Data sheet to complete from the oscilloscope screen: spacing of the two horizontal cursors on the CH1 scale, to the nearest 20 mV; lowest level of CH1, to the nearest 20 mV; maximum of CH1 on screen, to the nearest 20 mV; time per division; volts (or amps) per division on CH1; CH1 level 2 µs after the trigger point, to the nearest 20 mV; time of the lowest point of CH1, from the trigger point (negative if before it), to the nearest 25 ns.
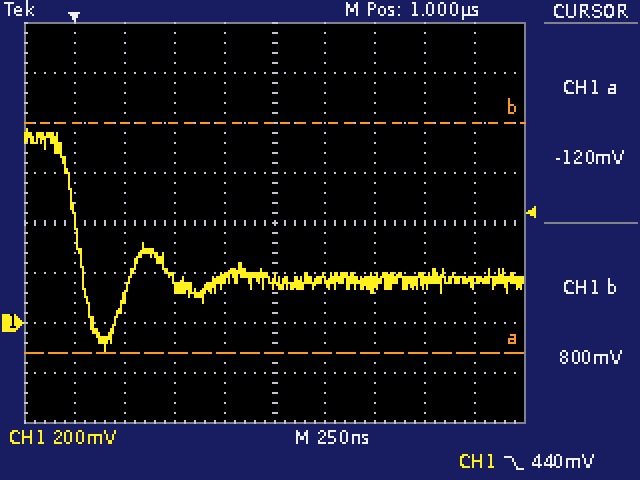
920 mV
-120 mV
780 mV
250 ns
200 mV
160 mV
+150 ns
